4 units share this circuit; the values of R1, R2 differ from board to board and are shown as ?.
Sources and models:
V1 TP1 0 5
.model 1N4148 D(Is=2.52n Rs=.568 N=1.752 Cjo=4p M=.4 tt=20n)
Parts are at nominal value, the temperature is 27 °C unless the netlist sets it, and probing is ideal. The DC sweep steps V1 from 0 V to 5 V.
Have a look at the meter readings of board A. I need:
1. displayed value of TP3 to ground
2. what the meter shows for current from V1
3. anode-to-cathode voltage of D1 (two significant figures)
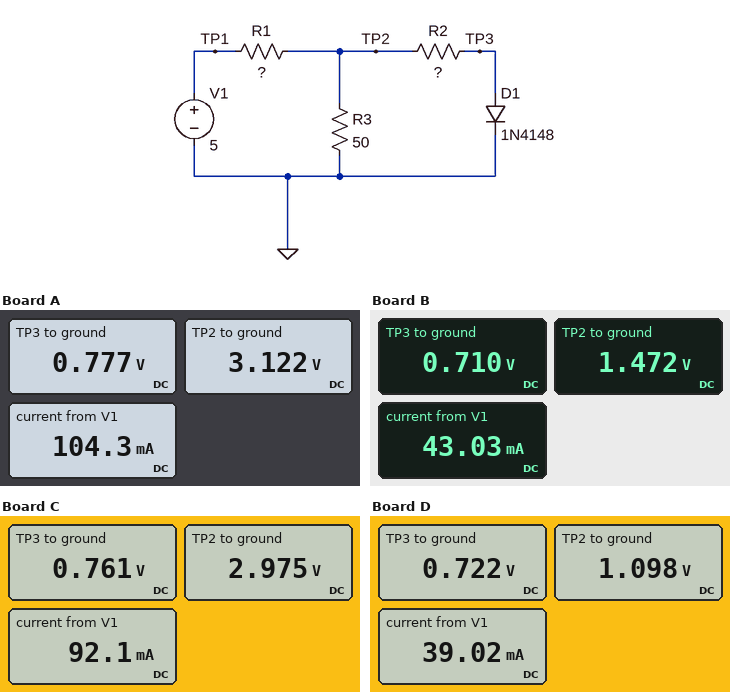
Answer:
0.777 V
104.3 mA
780 mV
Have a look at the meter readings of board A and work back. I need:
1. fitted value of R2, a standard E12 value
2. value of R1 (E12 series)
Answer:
56 Ω
18 Ω
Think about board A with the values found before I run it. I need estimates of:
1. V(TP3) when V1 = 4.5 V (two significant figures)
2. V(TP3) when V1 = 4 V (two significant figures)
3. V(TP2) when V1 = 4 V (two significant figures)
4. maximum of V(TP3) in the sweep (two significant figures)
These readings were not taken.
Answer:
770 mV
760 mV
2.5 V
780 mV
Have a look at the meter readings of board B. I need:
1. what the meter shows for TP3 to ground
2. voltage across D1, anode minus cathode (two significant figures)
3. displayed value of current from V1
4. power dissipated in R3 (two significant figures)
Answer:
0.710 V
710 mV
43.03 mA
43 mW
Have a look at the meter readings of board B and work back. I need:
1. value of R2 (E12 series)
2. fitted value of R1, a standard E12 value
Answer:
56 Ω
82 Ω
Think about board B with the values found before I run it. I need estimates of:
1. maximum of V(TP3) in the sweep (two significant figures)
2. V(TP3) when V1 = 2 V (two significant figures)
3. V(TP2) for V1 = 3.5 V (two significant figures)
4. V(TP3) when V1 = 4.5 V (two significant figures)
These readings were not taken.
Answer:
710 mV
610 mV
1.1 V
700 mV
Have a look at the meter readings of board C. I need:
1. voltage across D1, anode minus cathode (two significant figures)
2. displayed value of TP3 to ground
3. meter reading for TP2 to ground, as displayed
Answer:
760 mV
0.761 V
2.975 V
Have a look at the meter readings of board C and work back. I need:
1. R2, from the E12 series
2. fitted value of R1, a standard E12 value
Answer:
68 Ω
22 Ω
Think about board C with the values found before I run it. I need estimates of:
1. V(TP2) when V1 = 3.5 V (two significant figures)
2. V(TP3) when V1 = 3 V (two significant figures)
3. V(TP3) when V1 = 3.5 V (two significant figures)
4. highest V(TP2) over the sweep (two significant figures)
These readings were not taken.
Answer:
2.1 V
720 mV
730 mV
3.0 V
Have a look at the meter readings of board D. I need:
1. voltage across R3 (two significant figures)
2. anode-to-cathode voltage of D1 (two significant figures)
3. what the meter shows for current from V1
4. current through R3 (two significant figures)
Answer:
1.1 V
720 mV
39.02 mA
22 mA
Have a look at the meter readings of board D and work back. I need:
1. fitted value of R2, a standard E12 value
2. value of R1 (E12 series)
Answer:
22 Ω
100 Ω
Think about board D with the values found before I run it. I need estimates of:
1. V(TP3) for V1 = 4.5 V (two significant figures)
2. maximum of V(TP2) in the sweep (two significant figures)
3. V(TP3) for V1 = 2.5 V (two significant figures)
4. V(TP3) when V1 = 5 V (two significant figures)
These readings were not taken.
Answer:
710 mV
1.1 V
640 mV
720 mV
